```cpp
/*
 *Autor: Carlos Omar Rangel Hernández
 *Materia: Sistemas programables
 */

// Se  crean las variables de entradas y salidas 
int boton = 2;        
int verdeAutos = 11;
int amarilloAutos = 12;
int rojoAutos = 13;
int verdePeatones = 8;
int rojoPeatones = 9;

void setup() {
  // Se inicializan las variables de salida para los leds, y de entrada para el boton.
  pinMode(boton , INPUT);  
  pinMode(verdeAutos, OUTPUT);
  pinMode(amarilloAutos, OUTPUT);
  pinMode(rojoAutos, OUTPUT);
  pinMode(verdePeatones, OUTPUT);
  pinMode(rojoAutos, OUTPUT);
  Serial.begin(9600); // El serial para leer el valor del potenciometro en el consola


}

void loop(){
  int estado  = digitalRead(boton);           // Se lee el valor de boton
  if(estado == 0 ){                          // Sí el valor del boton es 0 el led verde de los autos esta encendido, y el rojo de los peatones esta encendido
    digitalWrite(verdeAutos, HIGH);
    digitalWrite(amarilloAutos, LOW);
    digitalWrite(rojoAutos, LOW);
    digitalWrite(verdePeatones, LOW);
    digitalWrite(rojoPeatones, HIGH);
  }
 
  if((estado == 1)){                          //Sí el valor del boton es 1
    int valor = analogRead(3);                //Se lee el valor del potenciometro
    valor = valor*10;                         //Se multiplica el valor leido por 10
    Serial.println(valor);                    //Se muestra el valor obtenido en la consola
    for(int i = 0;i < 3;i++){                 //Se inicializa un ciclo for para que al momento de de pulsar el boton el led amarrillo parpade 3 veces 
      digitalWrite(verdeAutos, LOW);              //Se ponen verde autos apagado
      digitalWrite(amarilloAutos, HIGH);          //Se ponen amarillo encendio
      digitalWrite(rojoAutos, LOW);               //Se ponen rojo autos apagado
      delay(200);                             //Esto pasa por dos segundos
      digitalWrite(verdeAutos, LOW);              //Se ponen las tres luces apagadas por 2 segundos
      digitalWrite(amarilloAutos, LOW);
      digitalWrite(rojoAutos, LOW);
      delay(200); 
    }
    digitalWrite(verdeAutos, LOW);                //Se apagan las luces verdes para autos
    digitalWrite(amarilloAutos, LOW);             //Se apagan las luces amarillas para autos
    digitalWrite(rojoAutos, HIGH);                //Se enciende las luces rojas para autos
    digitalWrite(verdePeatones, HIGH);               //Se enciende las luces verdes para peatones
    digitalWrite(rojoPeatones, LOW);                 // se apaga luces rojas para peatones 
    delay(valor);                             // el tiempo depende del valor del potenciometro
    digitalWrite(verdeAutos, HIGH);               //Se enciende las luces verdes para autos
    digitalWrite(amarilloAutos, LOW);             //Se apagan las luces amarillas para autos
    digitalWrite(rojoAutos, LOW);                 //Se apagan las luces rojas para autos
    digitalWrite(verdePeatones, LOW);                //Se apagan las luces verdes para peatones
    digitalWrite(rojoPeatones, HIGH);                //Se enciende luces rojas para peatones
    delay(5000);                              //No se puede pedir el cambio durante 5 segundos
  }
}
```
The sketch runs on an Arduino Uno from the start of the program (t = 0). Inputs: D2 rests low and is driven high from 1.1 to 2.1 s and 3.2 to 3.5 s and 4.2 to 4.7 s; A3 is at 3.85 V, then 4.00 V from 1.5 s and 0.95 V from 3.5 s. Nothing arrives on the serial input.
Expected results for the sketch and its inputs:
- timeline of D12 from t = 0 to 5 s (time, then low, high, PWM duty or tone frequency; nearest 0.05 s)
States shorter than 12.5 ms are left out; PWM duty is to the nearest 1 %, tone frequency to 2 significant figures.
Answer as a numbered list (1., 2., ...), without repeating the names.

1. 0 s low; 1.1 s high; 1.3 s low; 1.5 s high; 1.7 s low; 1.9 s high; 2.1 s low
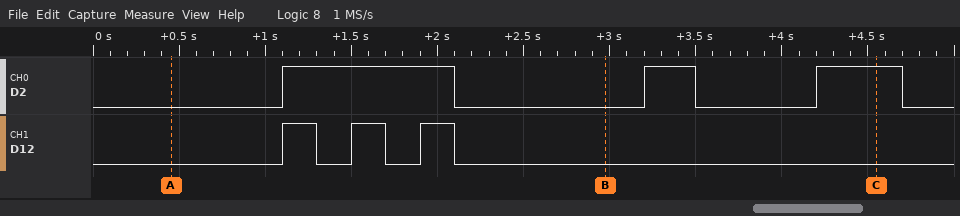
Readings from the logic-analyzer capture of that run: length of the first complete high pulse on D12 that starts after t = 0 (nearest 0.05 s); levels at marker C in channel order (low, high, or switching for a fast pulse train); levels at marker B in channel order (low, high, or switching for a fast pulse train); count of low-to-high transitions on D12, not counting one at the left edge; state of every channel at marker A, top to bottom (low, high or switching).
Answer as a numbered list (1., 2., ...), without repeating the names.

1. 0.20 s
2. D2 high, D12 low
3. D2 low, D12 low
4. 3
5. D2 low, D12 low
